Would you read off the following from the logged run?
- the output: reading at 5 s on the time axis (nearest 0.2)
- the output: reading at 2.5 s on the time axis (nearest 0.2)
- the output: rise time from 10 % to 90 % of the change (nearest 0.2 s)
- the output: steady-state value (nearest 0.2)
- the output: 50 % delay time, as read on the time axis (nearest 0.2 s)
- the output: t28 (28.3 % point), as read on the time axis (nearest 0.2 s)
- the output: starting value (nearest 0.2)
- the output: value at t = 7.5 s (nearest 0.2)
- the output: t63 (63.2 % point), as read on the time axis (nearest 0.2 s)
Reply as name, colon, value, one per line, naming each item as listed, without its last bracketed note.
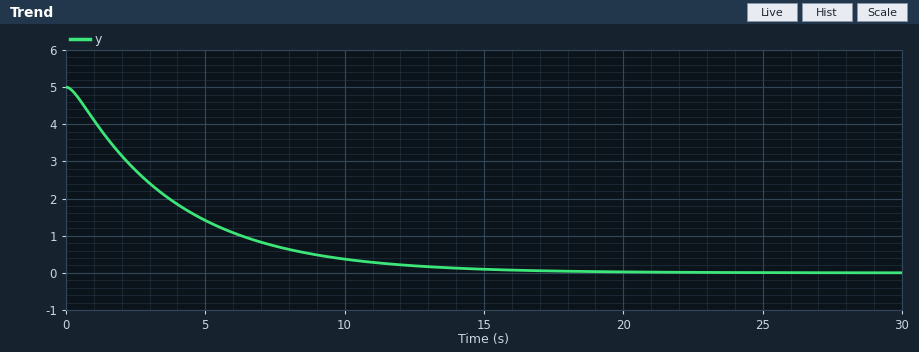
the output: reading at 5 s on the time axis: 1.4
the output: reading at 2.5 s on the time axis: 2.8
the output: rise time from 10 % to 90 % of the change: 8.2 s
the output: steady-state value: 0.0
the output: 50 % delay time, as read on the time axis: 2.8 s
the output: t28 (28.3 % point), as read on the time axis: 1.6 s
the output: starting value: 5.0
the output: value at t = 7.5 s: 0.8
the output: t63 (63.2 % point), as read on the time axis: 4.0 s
